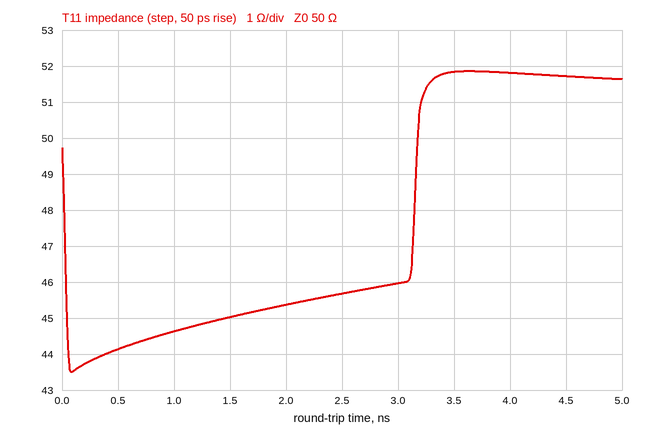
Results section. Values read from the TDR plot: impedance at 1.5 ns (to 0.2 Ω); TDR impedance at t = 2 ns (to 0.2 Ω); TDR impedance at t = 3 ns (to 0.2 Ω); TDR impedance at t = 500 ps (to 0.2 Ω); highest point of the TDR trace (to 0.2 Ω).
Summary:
45.0 Ω
45.4 Ω
46.0 Ω
44.2 Ω
51.8 Ω
